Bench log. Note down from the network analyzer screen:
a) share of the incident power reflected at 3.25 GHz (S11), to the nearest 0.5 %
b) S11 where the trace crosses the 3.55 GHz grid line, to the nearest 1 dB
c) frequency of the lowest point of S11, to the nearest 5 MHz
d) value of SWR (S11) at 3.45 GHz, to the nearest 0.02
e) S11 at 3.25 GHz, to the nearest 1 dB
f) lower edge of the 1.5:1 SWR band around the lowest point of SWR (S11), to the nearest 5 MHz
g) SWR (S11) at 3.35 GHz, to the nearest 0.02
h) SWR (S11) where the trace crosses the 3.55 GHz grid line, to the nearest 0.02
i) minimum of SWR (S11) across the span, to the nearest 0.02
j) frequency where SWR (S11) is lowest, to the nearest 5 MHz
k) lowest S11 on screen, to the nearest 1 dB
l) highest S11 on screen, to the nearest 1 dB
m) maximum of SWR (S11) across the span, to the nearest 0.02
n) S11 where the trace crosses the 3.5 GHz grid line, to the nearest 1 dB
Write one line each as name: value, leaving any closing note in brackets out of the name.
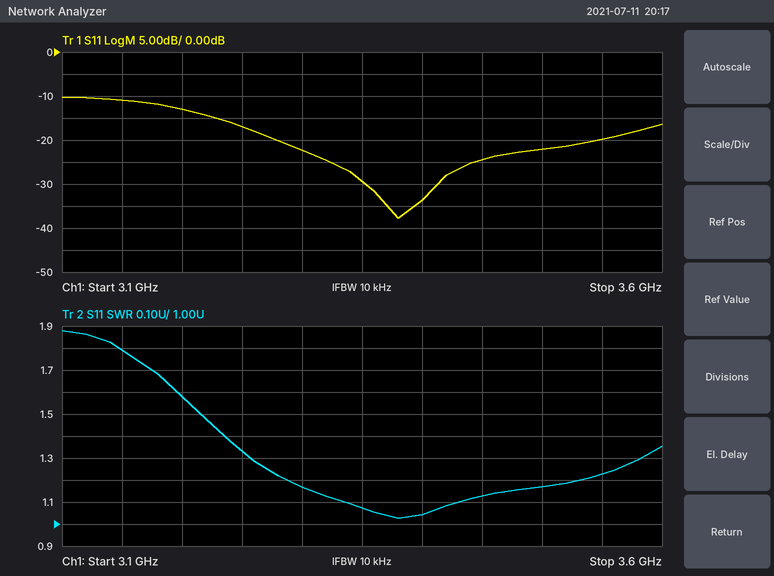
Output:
share of the incident power reflected at 3.25 GHz (S11), to the nearest 0.5 %: 2.0 %
S11 where the trace crosses the 3.55 GHz grid line, to the nearest 1 dB: -20 dB
frequency of the lowest point of S11, to the nearest 5 MHz: 3.380 GHz
value of SWR (S11) at 3.45 GHz, to the nearest 0.02: 1.12
S11 at 3.25 GHz, to the nearest 1 dB: -17 dB
lower edge of the 1.5:1 SWR band around the lowest point of SWR (S11), to the nearest 5 MHz: 3.215 GHz
SWR (S11) at 3.35 GHz, to the nearest 0.02: 1.08
SWR (S11) where the trace crosses the 3.55 GHz grid line, to the nearest 0.02: 1.22
minimum of SWR (S11) across the span, to the nearest 0.02: 1.02
frequency where SWR (S11) is lowest, to the nearest 5 MHz: 3.380 GHz
lowest S11 on screen, to the nearest 1 dB: -38 dB
highest S11 on screen, to the nearest 1 dB: -10 dB
maximum of SWR (S11) across the span, to the nearest 0.02: 1.88
S11 where the trace crosses the 3.5 GHz grid line, to the nearest 1 dB: -22 dB
